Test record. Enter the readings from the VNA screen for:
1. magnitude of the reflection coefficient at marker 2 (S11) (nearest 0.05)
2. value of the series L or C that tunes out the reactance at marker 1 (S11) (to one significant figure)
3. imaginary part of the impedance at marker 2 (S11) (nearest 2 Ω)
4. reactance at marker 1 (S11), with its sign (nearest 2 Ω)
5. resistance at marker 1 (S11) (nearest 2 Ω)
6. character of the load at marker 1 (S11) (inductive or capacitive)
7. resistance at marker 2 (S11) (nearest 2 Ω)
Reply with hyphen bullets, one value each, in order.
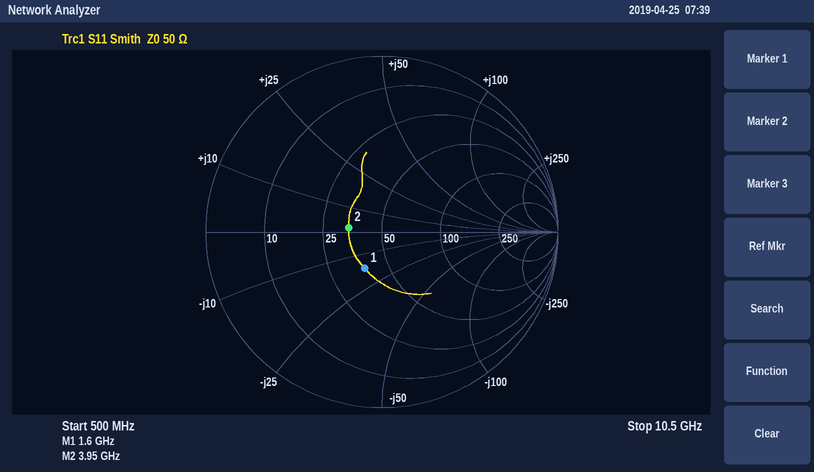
- 0.20
- 2 nH
- +2 Ω
- -16 Ω
- 38 Ω
- capacitive
- 34 Ω
